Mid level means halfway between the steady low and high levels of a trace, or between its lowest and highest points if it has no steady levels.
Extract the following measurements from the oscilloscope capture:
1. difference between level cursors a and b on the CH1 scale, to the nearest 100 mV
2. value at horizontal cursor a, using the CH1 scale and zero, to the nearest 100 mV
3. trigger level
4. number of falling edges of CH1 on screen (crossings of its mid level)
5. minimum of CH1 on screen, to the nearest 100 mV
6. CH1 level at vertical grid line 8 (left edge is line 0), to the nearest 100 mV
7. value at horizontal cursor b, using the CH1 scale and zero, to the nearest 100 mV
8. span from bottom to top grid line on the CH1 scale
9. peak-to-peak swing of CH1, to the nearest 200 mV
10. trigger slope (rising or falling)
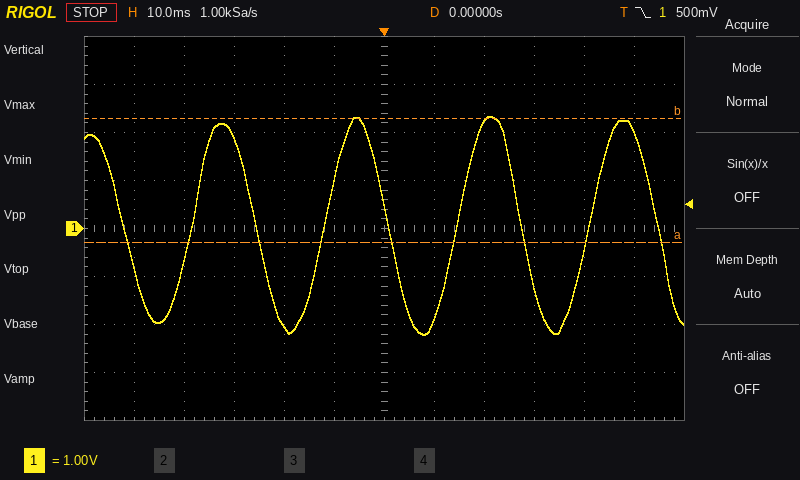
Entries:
2.6 V
-300 mV
500 mV
5
-2.2 V
2.2 V
2.3 V
8 V
4.6 V
falling
